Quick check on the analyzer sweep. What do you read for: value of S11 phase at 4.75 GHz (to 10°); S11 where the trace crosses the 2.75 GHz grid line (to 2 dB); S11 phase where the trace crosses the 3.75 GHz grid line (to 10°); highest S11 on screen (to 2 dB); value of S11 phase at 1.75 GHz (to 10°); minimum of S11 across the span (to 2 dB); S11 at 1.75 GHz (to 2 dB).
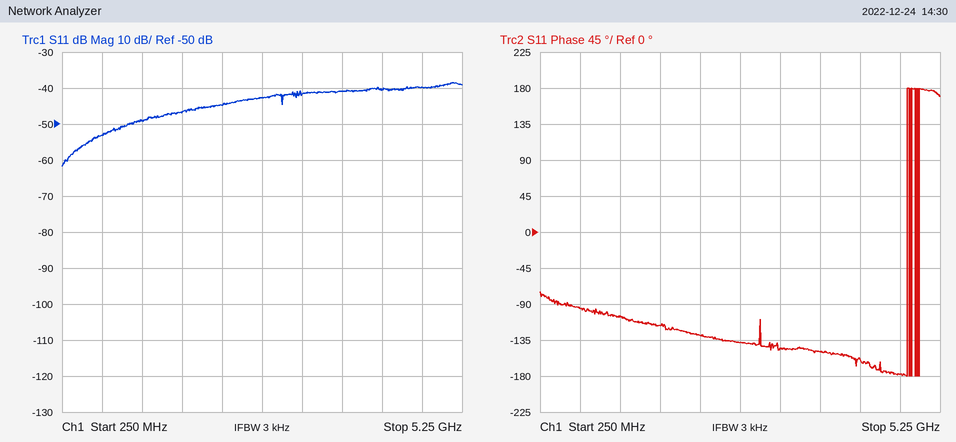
-180°
-42 dB
-150°
-38 dB
-120°
-62 dB
-46 dB
